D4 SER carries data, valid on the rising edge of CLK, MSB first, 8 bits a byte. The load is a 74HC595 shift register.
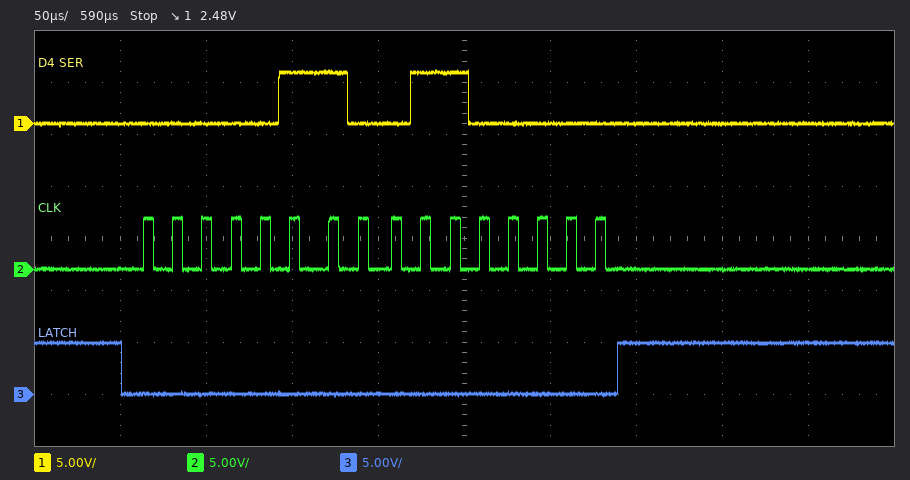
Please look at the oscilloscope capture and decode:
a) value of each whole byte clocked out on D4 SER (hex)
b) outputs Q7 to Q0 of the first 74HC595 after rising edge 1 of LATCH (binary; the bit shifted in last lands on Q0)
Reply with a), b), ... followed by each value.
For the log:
a) 06 60
b) 01100000
